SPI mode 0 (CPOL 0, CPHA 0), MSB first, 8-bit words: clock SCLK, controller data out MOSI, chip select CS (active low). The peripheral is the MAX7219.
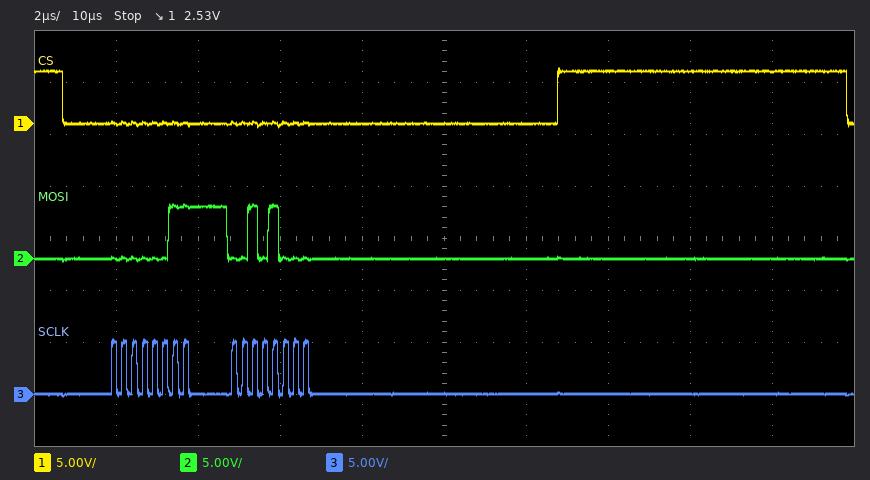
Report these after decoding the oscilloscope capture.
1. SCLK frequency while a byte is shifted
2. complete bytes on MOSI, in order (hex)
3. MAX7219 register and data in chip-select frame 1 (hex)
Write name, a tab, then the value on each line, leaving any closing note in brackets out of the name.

SCLK frequency while a byte is shifted	4 MHz
complete bytes on MOSI, in order	03 28
MAX7219 register and data in chip-select frame 1	register 0x3, data 0x28
